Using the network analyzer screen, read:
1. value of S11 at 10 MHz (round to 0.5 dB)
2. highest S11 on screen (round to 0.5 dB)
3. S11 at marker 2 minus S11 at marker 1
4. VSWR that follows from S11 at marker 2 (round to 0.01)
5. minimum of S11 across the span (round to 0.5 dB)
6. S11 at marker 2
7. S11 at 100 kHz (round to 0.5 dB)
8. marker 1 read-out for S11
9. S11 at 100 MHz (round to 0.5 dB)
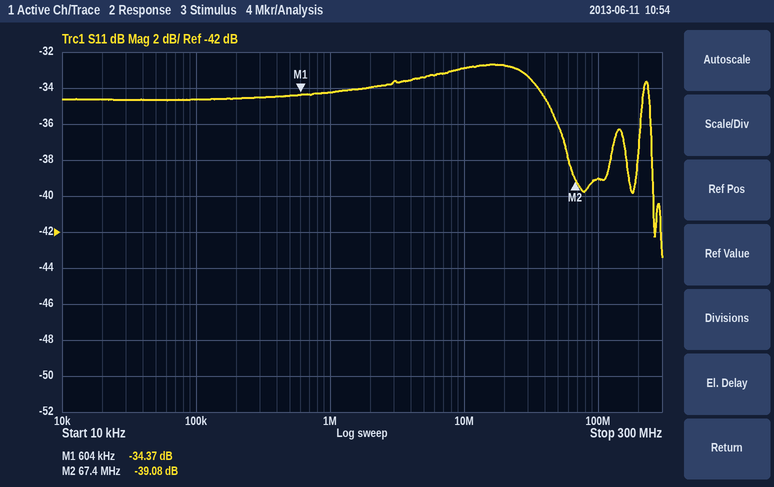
-33.0 dB
-32.5 dB
-4.71 dB
1.02
-43.5 dB
-39.08 dB
-34.5 dB
-34.37 dB
-39.0 dB
